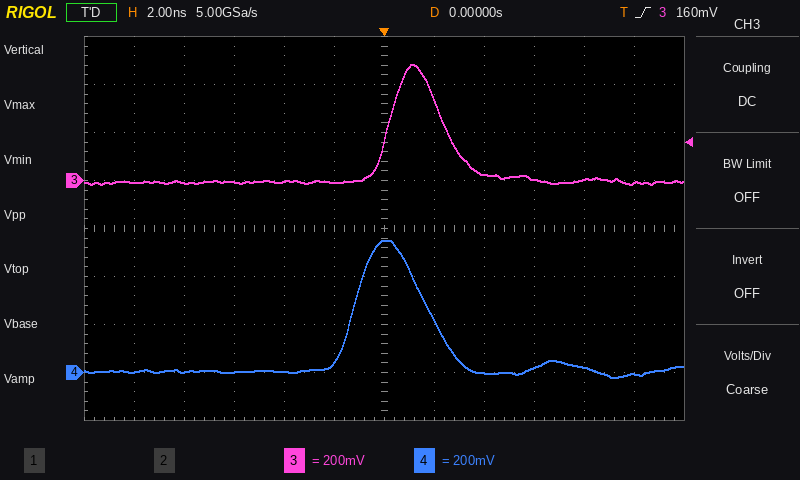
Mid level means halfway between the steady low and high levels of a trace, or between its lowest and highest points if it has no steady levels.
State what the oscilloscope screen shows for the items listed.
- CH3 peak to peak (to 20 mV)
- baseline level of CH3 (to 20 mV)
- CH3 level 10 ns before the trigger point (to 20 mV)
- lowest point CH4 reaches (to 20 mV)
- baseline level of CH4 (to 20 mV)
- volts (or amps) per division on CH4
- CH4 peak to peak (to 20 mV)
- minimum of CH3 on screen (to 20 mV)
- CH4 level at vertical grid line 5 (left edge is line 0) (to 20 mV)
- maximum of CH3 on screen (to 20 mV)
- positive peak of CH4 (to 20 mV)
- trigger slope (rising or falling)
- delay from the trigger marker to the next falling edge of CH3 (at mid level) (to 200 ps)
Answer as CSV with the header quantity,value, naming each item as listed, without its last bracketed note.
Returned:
quantity,value
CH3 peak to peak,500 mV
baseline level of CH3,0 mV
CH3 level 10 ns before the trigger point,0 mV
lowest point CH4 reaches,-20 mV
baseline level of CH4,0 mV
volts (or amps) per division on CH4,200 mV
CH4 peak to peak,580 mV
minimum of CH3 on screen,-20 mV
CH4 level at vertical grid line 5 (left edge is line 0),40 mV
maximum of CH3 on screen,480 mV
positive peak of CH4,560 mV
trigger slope,rising
delay from the trigger marker to the next falling edge of CH3 (at mid level),2.4 ns
